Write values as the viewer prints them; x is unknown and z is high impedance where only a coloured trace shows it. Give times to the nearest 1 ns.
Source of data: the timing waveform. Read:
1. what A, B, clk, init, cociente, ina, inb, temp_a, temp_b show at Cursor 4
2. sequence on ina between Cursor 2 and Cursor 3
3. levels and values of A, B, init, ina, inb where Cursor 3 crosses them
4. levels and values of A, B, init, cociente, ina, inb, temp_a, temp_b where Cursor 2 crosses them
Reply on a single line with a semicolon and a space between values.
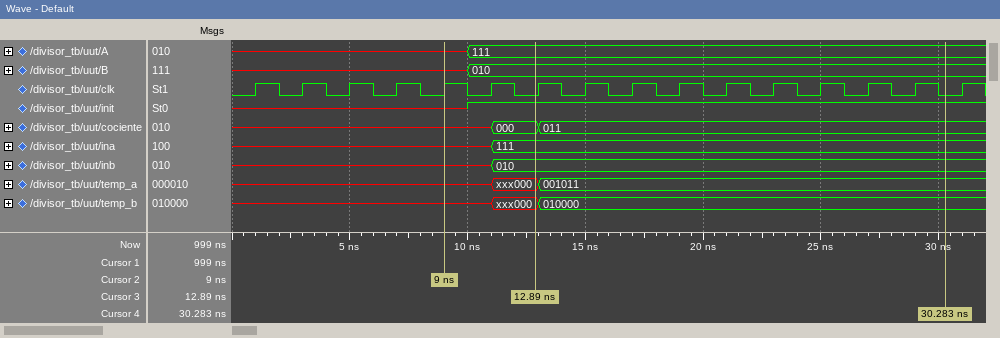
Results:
A=111, B=010, clk=0, init=1, cociente=011, ina=111, inb=010, temp_a=001011, temp_b=010000; x, 111; A=111, B=010, init=1, ina=111, inb=010; A=x, B=x, init=x, cociente=x, ina=x, inb=x, temp_a=x, temp_b=x
